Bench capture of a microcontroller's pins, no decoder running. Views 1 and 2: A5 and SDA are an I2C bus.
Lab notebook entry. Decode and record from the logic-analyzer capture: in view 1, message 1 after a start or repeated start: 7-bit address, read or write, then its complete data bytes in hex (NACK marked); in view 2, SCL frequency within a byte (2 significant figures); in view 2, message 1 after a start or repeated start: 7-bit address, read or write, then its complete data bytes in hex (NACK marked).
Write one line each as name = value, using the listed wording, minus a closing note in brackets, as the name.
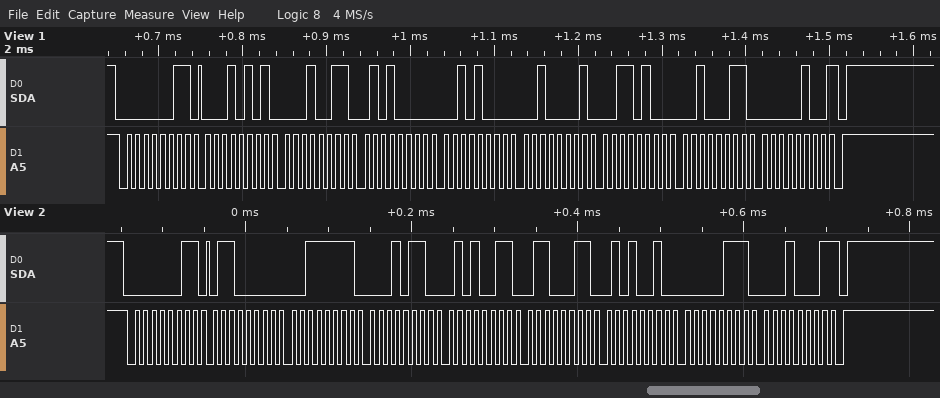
in view 1, message 1 after a start or repeated start: 7-bit address, read or write, then its complete data bytes in hex = 0x01 read: 15 13 50 28 21 34 23 04 NACK
in view 2, SCL frequency within a byte = 100 kHz
in view 2, message 1 after a start or repeated start: 7-bit address, read or write, then its complete data bytes in hex = 0x01 read: 60 3F 16 53 63 52 07 11 NACK
